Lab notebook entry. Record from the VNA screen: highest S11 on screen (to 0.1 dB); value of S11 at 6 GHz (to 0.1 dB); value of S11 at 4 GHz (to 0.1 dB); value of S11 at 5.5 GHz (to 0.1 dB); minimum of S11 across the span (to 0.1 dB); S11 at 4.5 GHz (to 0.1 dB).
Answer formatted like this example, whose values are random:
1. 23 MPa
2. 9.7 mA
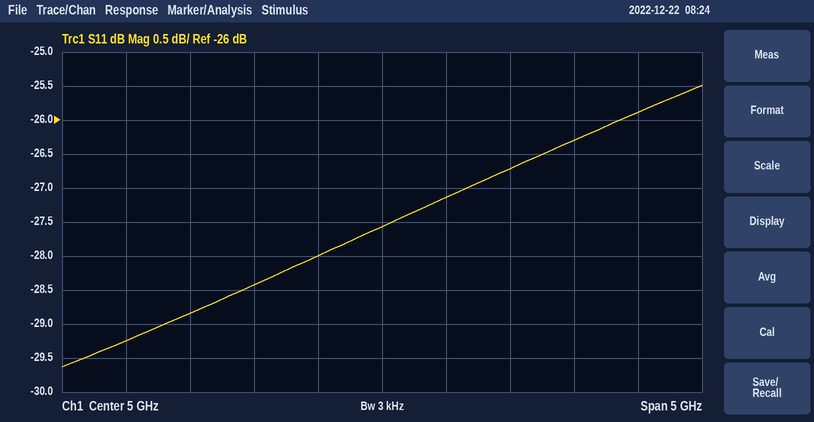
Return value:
1. -25.5 dB
2. -26.7 dB
3. -28.4 dB
4. -27.1 dB
5. -29.6 dB
6. -28.0 dB
